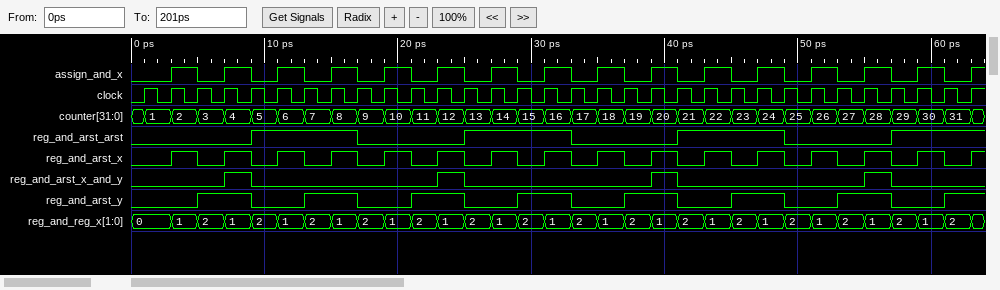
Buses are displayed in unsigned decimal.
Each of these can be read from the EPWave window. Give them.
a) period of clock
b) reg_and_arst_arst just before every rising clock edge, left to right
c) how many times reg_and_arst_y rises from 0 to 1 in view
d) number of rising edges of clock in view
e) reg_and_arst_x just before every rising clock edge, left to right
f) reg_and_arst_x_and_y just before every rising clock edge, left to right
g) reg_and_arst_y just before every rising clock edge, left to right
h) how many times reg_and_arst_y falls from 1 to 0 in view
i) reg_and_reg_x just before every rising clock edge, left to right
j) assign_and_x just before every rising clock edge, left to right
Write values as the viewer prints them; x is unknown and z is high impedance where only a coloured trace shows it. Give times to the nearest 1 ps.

2 ps
0 0 0 0 0 1 1 1 1 0 0 0 0 1 1 1 1 0 0 0 0 1 1 1 1 0 0 0 0 1 1 1
8
32
0 0 1 0 1 0 1 0 1 0 1 0 1 0 1 0 1 0 1 0 1 0 1 0 1 0 1 0 1 0 1 0
0 0 0 0 1 0 0 0 0 0 0 0 1 0 0 0 0 0 0 0 1 0 0 0 0 0 0 0 1 0 0 0
0 0 0 1 1 0 0 1 1 0 0 1 1 0 0 1 1 0 0 1 1 0 0 1 1 0 0 1 1 0 0 1
7
0, 0, 1, 2, 1, 2, 1, 2, 1, 2, 1, 2, 1, 2, 1, 2, 1, 2, 1, 2, 1, 2, 1, 2, 1, 2, 1, 2, 1, 2, 1, 2
0 0 1 0 1 0 1 0 1 0 1 0 1 0 1 0 1 0 1 0 1 0 1 0 1 0 1 0 1 0 1 0
